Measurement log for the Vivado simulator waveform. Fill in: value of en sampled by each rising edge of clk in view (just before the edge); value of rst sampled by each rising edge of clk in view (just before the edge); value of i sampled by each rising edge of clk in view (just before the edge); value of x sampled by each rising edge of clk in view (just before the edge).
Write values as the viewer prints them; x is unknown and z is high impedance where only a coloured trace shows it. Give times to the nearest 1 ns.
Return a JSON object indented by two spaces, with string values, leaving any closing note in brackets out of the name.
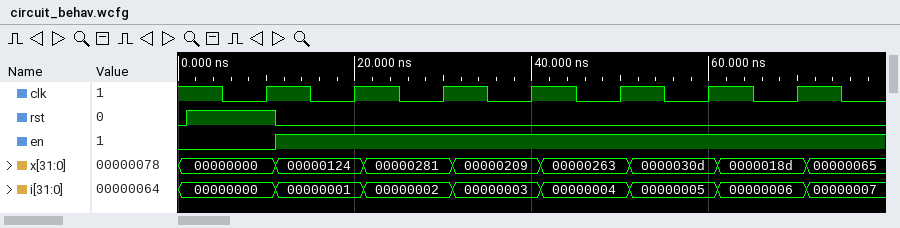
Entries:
{
  "value of en sampled by each rising edge of clk in view": "0 1 1 1 1 1 1",
  "value of rst sampled by each rising edge of clk in view": "1 0 0 0 0 0 0",
  "value of i sampled by each rising edge of clk in view": "00000000, 00000001, 00000002, 00000003, 00000004, 00000005, 00000006",
  "value of x sampled by each rising edge of clk in view": "00000000, 00000124, 00000281, 00000209, 00000263, 0000030d, 0000018d"
}
